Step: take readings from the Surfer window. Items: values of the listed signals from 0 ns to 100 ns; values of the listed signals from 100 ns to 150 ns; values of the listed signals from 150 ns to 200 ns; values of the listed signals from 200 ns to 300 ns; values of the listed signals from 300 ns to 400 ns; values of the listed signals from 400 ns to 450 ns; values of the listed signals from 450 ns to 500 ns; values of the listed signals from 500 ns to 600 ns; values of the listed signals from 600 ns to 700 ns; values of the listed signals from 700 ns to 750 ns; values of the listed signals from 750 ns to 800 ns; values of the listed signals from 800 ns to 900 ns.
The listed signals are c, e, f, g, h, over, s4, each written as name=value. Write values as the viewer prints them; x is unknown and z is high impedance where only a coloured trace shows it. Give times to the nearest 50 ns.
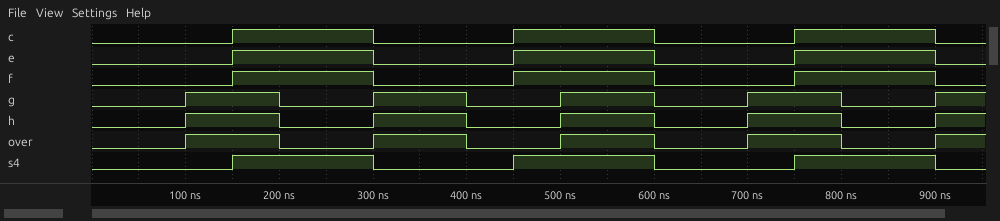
c=0, e=0, f=0, g=0, h=0, over=0, s4=0
c=0, e=0, f=0, g=1, h=1, over=1, s4=0
c=1, e=1, f=1, g=1, h=1, over=1, s4=1
c=1, e=1, f=1, g=0, h=0, over=0, s4=1
c=0, e=0, f=0, g=1, h=1, over=1, s4=0
c=0, e=0, f=0, g=0, h=0, over=0, s4=0
c=1, e=1, f=1, g=0, h=0, over=0, s4=1
c=1, e=1, f=1, g=1, h=1, over=1, s4=1
c=0, e=0, f=0, g=0, h=0, over=0, s4=0
c=0, e=0, f=0, g=1, h=1, over=1, s4=0
c=1, e=1, f=1, g=1, h=1, over=1, s4=1
c=1, e=1, f=1, g=0, h=0, over=0, s4=1
